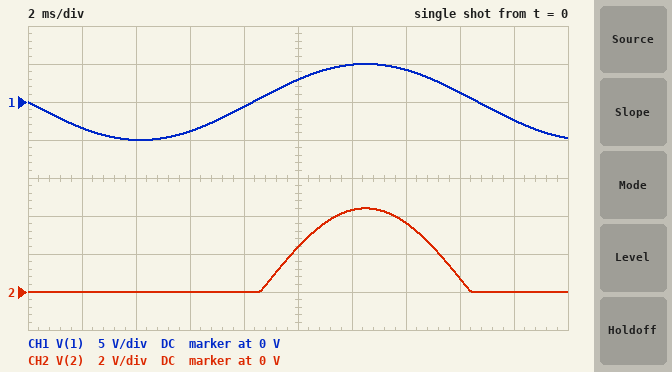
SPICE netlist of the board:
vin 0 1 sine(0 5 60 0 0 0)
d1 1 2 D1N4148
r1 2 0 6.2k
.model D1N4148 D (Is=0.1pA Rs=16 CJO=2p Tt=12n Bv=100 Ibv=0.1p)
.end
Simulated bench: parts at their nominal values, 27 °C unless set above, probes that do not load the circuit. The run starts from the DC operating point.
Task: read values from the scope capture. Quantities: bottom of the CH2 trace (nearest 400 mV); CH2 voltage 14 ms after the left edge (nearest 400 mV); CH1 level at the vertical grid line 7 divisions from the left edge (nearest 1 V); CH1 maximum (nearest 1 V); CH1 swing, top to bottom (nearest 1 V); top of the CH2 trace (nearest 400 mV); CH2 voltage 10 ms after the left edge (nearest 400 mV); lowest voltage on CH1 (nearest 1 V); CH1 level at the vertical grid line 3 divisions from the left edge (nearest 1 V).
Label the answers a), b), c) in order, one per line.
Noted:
a) 0 V
b) 3.6 V
c) 4 V
d) 5 V
e) 10 V
f) 4.4 V
g) 2.4 V
h) -5 V
i) -4 V
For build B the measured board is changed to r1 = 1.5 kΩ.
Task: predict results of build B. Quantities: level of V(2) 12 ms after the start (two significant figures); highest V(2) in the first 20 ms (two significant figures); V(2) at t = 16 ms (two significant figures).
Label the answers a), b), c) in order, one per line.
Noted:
a) 4.2 V
b) 4.3 V
c) 660 mV
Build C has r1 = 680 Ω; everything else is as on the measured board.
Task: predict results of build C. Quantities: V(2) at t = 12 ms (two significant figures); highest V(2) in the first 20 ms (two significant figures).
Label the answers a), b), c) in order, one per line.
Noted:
a) 4.2 V
b) 4.3 V
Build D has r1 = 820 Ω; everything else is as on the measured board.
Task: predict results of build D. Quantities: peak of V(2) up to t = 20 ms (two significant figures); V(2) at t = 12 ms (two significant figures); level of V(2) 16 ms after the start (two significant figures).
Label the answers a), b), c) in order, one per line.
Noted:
a) 4.3 V
b) 4.2 V
c) 640 mV
